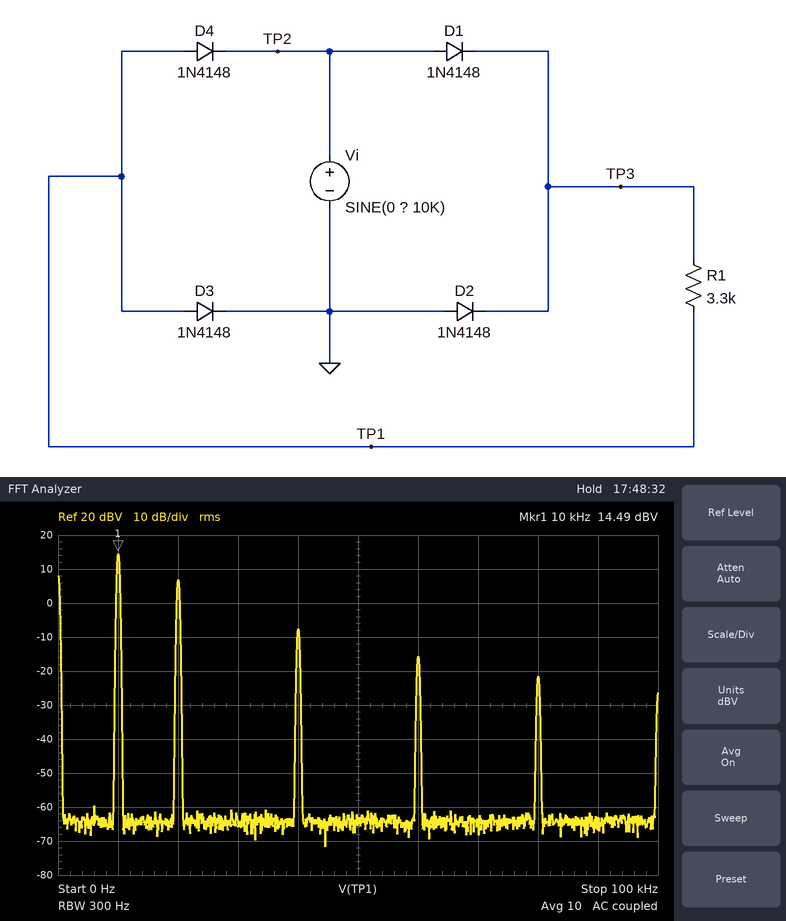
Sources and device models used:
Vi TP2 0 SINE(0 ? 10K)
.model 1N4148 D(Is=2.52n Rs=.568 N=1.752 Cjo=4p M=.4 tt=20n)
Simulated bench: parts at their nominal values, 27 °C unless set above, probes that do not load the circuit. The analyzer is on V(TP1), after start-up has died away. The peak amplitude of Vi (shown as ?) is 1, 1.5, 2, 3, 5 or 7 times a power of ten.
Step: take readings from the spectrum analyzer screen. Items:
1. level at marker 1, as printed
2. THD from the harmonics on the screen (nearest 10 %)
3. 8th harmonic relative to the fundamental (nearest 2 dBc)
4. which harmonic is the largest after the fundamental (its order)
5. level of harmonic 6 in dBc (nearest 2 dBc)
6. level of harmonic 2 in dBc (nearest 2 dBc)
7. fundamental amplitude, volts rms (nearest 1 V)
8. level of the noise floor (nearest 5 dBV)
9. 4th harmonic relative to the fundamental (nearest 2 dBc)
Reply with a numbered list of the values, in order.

1. 14.49 dBV
2. 40 %
3. -36 dBc
4. 2
5. -30 dBc
6. -8 dBc
7. 5 V
8. -65 dBV
9. -22 dBc
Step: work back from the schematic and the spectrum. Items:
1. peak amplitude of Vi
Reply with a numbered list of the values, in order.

1. 15 V
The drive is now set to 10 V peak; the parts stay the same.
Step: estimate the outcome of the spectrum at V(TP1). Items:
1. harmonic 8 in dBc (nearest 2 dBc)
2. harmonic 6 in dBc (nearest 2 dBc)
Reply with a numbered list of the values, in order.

1. -38 dBc
2. -32 dBc
